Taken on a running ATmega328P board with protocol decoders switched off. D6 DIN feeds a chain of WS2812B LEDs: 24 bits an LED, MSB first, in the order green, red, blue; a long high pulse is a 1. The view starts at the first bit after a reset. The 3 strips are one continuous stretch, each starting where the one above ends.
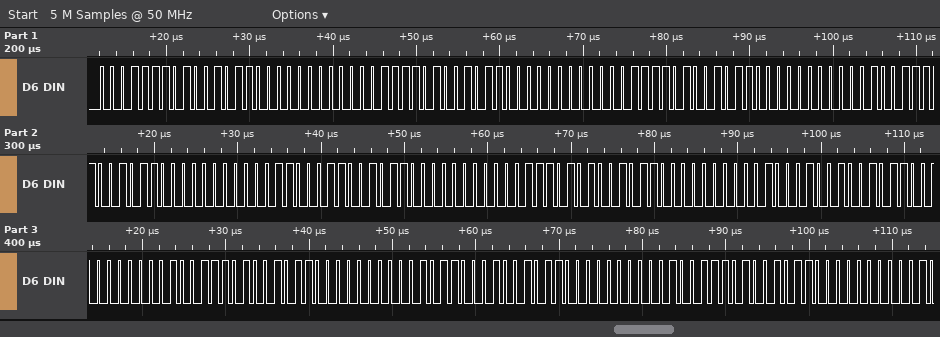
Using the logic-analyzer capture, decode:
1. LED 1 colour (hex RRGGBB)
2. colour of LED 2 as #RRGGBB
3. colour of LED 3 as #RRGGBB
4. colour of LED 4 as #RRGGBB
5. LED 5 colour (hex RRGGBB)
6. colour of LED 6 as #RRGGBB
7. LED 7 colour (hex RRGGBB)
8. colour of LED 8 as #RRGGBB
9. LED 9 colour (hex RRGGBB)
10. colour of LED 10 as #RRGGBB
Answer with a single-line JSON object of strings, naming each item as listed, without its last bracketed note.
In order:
{"LED 1 colour": "#961E00", "colour of LED 2 as #RRGGBB": "#961E00", "colour of LED 3 as #RRGGBB": "#961E00", "colour of LED 4 as #RRGGBB": "#962700", "LED 5 colour": "#963100", "colour of LED 6 as #RRGGBB": "#963A00", "LED 7 colour": "#964400", "colour of LED 8 as #RRGGBB": "#964E00", "LED 9 colour": "#965800", "colour of LED 10 as #RRGGBB": "#964E00"}
